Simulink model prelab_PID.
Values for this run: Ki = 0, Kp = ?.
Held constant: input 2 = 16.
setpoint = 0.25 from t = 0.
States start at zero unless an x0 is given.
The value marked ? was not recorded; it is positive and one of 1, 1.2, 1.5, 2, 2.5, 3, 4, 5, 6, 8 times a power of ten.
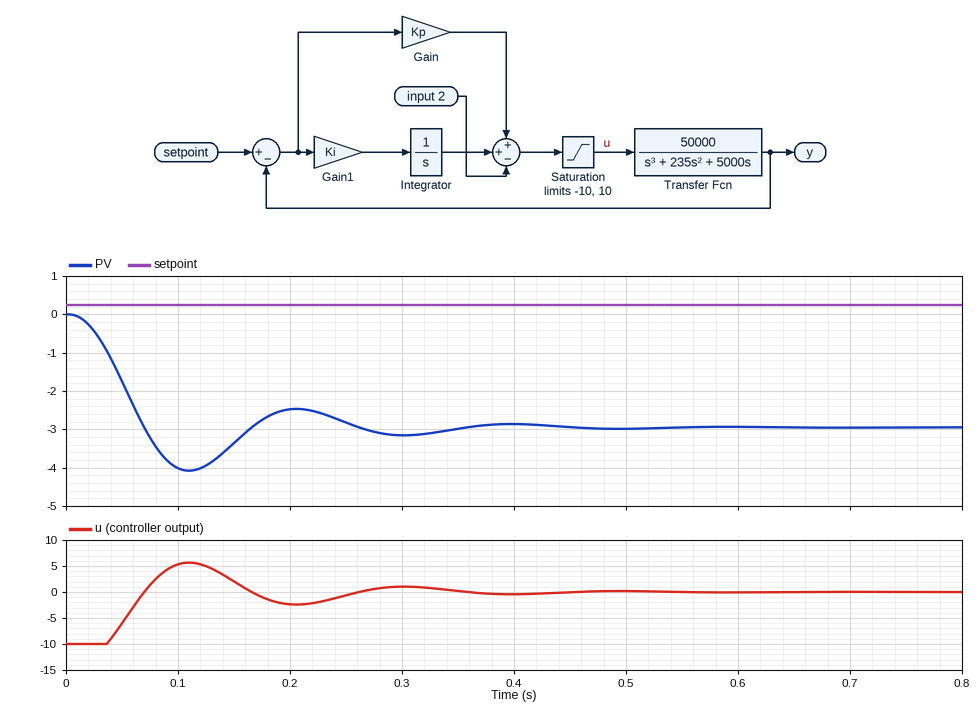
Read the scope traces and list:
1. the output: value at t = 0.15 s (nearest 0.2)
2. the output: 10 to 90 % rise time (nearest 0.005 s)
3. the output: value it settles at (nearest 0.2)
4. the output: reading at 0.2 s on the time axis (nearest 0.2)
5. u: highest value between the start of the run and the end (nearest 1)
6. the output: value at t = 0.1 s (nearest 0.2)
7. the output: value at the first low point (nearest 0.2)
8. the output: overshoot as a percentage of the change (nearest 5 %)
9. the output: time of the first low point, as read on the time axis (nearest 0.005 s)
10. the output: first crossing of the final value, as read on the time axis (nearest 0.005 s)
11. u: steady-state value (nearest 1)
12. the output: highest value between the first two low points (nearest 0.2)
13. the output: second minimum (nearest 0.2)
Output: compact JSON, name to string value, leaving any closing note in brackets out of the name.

{"the output: value at t = 0.15 s": "-3.4", "the output: 10 to 90 % rise time": "0.045 s", "the output: value it settles at": "-3.0", "the output: reading at 0.2 s on the time axis": "-2.4", "u: highest value between the start of the run and the end": "6", "the output: value at t = 0.1 s": "-4.0", "the output: value at the first low point": "-4.0", "the output: overshoot as a percentage of the change": "40 %", "the output: time of the first low point, as read on the time axis": "0.110 s", "the output: first crossing of the final value, as read on the time axis": "0.070 s", "u: steady-state value": "0", "the output: highest value between the first two low points": "-2.4", "the output: second minimum": "-3.2"}
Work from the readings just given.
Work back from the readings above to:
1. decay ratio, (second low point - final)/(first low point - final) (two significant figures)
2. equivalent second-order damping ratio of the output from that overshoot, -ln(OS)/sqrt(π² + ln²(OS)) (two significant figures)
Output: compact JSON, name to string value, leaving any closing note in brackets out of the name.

{"decay ratio, (second low point - final)/(first low point - final)": "0.20", "equivalent second-order damping ratio of the output from that overshoot, -ln(OS)/sqrt(π² + ln²(OS))": "0.28"}
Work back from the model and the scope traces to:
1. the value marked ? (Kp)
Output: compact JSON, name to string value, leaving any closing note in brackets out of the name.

{"the value marked ?": "5"}
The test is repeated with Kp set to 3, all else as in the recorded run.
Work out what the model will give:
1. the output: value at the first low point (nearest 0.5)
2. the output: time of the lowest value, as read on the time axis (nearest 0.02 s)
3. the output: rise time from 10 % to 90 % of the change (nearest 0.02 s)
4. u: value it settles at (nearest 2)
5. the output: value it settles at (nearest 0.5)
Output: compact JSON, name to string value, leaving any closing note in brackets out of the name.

{"the output: value at the first low point": "-6.5", "the output: time of the lowest value, as read on the time axis": "0.14 s", "the output: rise time from 10 % to 90 % of the change": "0.06 s", "u: value it settles at": "0", "the output: value it settles at": "-5.0"}
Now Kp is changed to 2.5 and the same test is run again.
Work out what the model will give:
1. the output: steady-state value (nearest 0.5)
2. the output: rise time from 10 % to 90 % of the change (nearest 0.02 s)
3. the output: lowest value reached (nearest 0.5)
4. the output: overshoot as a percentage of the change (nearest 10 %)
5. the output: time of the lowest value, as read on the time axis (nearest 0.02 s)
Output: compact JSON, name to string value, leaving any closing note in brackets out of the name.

{"the output: steady-state value": "-6.0", "the output: rise time from 10 % to 90 % of the change": "0.08 s", "the output: lowest value reached": "-7.5", "the output: overshoot as a percentage of the change": "20 %", "the output: time of the lowest value, as read on the time axis": "0.16 s"}
